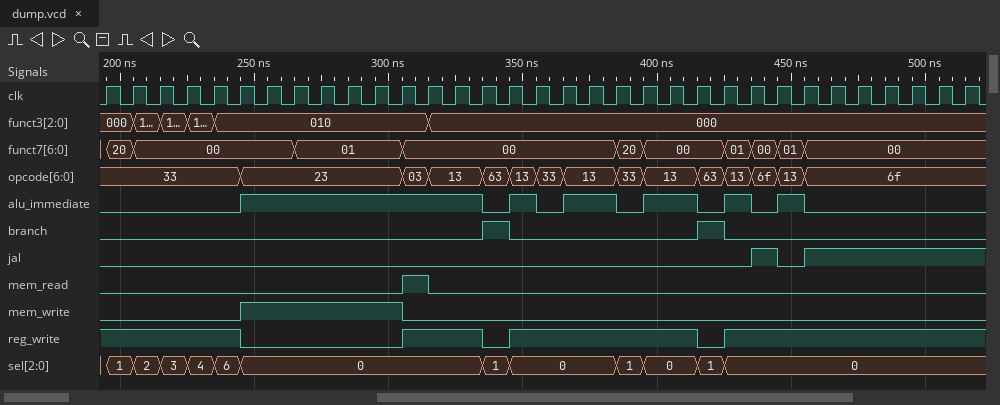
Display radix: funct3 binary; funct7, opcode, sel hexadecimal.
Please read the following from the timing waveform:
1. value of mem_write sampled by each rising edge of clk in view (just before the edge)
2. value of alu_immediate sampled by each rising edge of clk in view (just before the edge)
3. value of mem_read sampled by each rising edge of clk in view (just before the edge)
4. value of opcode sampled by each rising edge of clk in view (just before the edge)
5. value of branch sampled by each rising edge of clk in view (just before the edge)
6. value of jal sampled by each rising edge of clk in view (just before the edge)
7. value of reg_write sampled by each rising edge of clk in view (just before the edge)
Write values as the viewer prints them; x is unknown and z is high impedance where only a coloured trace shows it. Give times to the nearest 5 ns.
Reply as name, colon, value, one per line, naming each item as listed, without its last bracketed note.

value of mem_write sampled by each rising edge of clk in view: 0 0 0 0 0 0 1 1 1 1 1 1 0 0 0 0 0 0 0 0 0 0 0 0 0 0 0 0 0 0 0 0 0
value of alu_immediate sampled by each rising edge of clk in view: 0 0 0 0 0 0 1 1 1 1 1 1 1 1 1 0 1 0 1 1 0 1 1 0 1 0 1 0 0 0 0 0 0
value of mem_read sampled by each rising edge of clk in view: 0 0 0 0 0 0 0 0 0 0 0 0 1 0 0 0 0 0 0 0 0 0 0 0 0 0 0 0 0 0 0 0 0
value of opcode sampled by each rising edge of clk in view: 33, 33, 33, 33, 33, 33, 23, 23, 23, 23, 23, 23, 03, 13, 13, 63, 13, 33, 13, 13, 33, 13, 13, 63, 13, 6f, 13, 6f, 6f, 6f, 6f, 6f, 6f
value of branch sampled by each rising edge of clk in view: 0 0 0 0 0 0 0 0 0 0 0 0 0 0 0 1 0 0 0 0 0 0 0 1 0 0 0 0 0 0 0 0 0
value of jal sampled by each rising edge of clk in view: 0 0 0 0 0 0 0 0 0 0 0 0 0 0 0 0 0 0 0 0 0 0 0 0 0 1 0 1 1 1 1 1 1
value of reg_write sampled by each rising edge of clk in view: 1 1 1 1 1 1 0 0 0 0 0 0 1 1 1 0 1 1 1 1 1 1 1 0 1 1 1 1 1 1 1 1 1
